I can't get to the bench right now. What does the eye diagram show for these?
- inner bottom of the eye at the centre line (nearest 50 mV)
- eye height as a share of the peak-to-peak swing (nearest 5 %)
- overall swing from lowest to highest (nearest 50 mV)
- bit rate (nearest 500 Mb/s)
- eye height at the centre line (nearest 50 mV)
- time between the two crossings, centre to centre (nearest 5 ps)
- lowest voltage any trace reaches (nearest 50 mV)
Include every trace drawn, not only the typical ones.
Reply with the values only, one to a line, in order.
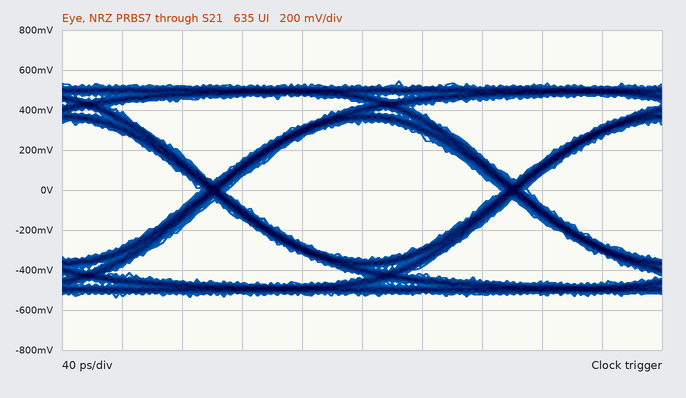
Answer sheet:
-350 mV
65 %
1.10 V
5.0 Gb/s
700 mV
200 ps
-550 mV
